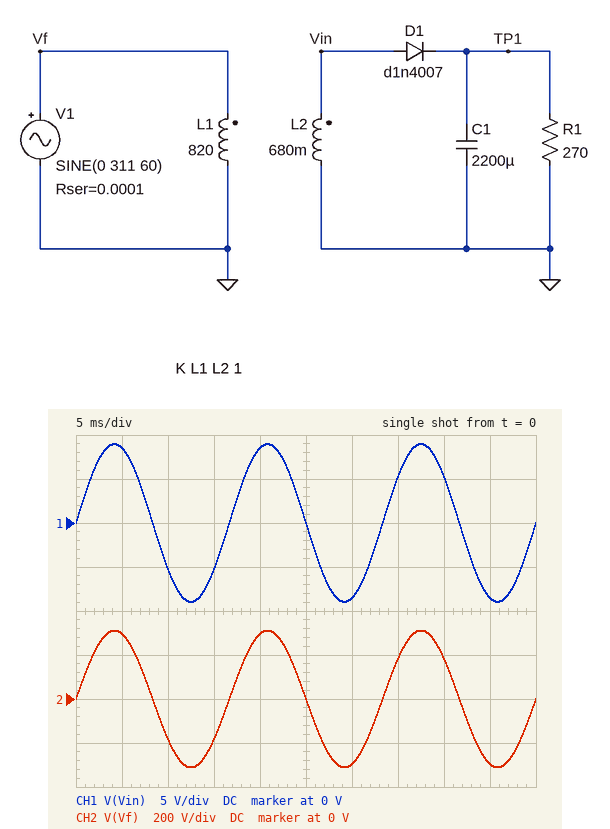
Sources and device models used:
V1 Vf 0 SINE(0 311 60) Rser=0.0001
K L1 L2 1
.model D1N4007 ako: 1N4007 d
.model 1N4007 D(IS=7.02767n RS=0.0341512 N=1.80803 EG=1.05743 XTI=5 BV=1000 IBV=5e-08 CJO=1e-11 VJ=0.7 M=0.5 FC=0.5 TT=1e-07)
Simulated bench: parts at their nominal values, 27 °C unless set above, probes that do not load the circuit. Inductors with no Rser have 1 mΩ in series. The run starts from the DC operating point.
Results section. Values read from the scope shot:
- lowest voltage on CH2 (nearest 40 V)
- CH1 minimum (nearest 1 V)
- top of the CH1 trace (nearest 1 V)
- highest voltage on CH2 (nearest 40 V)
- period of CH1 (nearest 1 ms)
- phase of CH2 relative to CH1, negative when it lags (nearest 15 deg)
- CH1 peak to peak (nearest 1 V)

-320 V
-9 V
9 V
320 V
17 ms
0 deg
18 V
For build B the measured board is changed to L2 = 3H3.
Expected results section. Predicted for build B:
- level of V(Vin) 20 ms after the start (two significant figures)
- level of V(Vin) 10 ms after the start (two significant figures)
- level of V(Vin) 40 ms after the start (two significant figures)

19 V
-12 V
12 V
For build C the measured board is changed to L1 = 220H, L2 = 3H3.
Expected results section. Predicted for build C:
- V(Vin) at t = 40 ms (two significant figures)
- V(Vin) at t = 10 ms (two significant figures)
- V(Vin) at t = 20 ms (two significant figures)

22 V
-22 V
36 V
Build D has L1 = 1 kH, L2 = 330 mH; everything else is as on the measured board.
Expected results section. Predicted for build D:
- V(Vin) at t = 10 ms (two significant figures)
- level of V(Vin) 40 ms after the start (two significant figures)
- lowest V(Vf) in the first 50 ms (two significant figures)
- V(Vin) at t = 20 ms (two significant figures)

-3.3 V
3.3 V
-310 V
5.4 V
